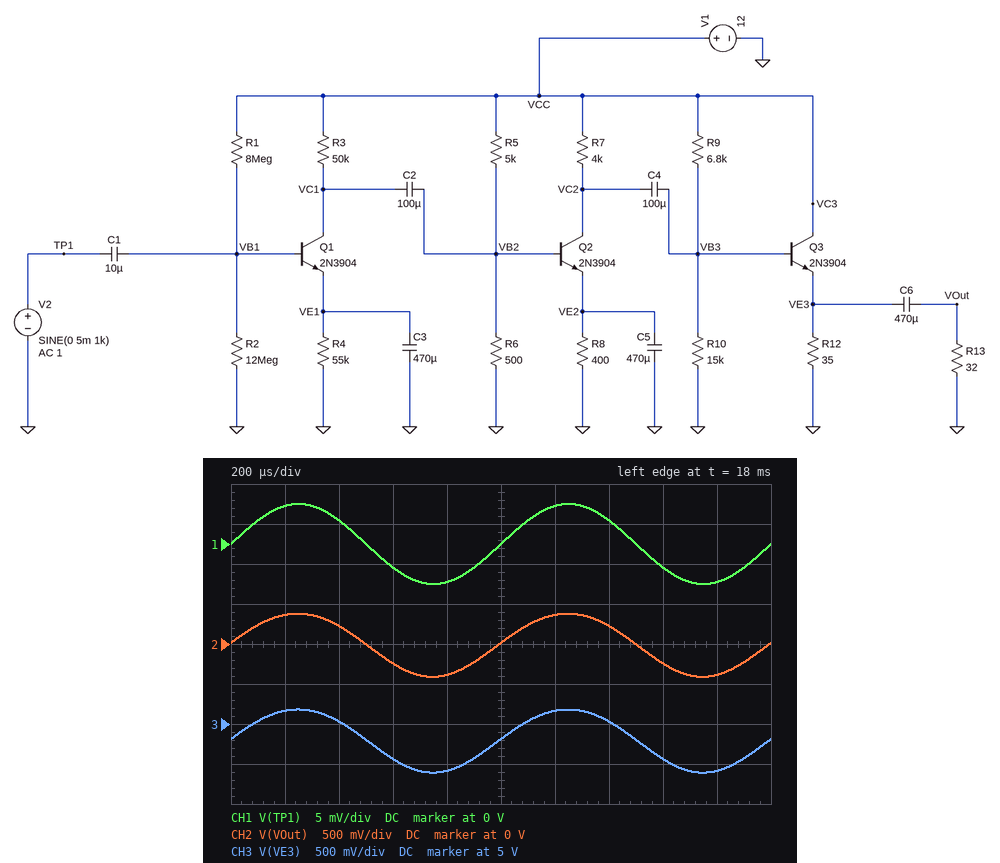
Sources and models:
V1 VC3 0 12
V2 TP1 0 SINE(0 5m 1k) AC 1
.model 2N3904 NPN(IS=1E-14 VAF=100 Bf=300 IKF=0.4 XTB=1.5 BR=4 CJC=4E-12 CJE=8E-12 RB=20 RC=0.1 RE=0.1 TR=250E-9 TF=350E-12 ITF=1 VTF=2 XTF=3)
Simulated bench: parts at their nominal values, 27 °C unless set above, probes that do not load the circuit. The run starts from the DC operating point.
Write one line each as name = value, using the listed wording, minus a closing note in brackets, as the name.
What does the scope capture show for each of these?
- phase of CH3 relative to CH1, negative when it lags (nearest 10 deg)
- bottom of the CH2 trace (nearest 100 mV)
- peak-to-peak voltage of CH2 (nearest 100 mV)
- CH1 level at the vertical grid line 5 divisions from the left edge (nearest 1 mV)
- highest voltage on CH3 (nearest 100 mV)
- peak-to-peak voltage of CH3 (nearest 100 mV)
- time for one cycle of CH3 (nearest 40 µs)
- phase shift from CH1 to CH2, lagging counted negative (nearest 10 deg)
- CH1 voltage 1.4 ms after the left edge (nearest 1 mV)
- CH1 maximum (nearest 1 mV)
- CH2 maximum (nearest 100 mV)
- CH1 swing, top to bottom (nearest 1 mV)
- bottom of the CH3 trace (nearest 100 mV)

phase of CH3 relative to CH1, negative when it lags = 0 deg
bottom of the CH2 trace = -400 mV
peak-to-peak voltage of CH2 = 800 mV
CH1 level at the vertical grid line 5 divisions from the left edge = 0 V
highest voltage on CH3 = 5.2 V
peak-to-peak voltage of CH3 = 800 mV
time for one cycle of CH3 = 1.00 ms
phase shift from CH1 to CH2, lagging counted negative = 0 deg
CH1 voltage 1.4 ms after the left edge = 3 mV
CH1 maximum = 5 mV
CH2 maximum = 400 mV
CH1 swing, top to bottom = 10 mV
bottom of the CH3 trace = 4.4 V
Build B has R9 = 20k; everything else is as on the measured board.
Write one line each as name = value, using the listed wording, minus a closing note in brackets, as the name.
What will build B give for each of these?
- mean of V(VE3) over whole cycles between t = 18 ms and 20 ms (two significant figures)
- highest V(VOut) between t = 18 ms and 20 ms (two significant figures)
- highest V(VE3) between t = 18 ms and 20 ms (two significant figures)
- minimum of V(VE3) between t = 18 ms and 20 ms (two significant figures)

mean of V(VE3) over whole cycles between t = 18 ms and 20 ms = 2.3 V
highest V(VOut) between t = 18 ms and 20 ms = 480 mV
highest V(VE3) between t = 18 ms and 20 ms = 2.8 V
minimum of V(VE3) between t = 18 ms and 20 ms = 1.8 V
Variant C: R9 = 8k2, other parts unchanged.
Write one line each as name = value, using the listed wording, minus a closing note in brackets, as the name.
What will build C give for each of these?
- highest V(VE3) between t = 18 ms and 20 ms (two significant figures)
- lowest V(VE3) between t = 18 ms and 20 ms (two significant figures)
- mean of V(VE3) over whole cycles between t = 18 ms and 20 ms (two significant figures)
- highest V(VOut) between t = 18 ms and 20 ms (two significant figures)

highest V(VE3) between t = 18 ms and 20 ms = 4.7 V
lowest V(VE3) between t = 18 ms and 20 ms = 3.9 V
mean of V(VE3) over whole cycles between t = 18 ms and 20 ms = 4.3 V
highest V(VOut) between t = 18 ms and 20 ms = 400 mV
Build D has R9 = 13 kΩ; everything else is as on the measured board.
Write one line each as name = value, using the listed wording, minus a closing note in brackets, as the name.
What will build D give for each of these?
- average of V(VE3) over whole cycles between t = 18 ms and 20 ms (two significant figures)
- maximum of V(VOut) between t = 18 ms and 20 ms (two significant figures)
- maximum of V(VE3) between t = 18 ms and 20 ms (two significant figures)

average of V(VE3) over whole cycles between t = 18 ms and 20 ms = 3.2 V
maximum of V(VOut) between t = 18 ms and 20 ms = 440 mV
maximum of V(VE3) between t = 18 ms and 20 ms = 3.7 V
